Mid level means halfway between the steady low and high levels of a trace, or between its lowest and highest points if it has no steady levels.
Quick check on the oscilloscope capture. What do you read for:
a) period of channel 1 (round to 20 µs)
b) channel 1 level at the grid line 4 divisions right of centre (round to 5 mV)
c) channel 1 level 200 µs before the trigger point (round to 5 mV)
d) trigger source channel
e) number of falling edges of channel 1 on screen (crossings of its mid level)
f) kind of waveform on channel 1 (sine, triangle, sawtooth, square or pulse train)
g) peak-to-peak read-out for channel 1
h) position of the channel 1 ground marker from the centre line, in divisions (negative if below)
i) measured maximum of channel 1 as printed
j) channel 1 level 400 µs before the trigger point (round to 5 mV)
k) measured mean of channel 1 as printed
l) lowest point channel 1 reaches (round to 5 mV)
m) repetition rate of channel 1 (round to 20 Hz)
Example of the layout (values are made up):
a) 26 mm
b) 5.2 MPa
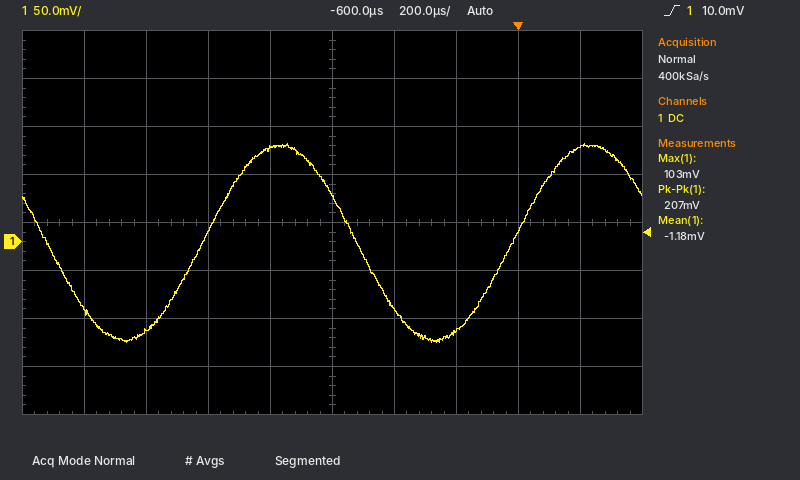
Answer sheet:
a) 1.00 ms
b) 100 mV
c) -95 mV
d) channel 1
e) 2
f) sine
g) 207 mV
h) -0.4 div
i) 103 mV
j) -70 mV
k) -1.18 mV
l) -105 mV
m) 1.00 kHz
